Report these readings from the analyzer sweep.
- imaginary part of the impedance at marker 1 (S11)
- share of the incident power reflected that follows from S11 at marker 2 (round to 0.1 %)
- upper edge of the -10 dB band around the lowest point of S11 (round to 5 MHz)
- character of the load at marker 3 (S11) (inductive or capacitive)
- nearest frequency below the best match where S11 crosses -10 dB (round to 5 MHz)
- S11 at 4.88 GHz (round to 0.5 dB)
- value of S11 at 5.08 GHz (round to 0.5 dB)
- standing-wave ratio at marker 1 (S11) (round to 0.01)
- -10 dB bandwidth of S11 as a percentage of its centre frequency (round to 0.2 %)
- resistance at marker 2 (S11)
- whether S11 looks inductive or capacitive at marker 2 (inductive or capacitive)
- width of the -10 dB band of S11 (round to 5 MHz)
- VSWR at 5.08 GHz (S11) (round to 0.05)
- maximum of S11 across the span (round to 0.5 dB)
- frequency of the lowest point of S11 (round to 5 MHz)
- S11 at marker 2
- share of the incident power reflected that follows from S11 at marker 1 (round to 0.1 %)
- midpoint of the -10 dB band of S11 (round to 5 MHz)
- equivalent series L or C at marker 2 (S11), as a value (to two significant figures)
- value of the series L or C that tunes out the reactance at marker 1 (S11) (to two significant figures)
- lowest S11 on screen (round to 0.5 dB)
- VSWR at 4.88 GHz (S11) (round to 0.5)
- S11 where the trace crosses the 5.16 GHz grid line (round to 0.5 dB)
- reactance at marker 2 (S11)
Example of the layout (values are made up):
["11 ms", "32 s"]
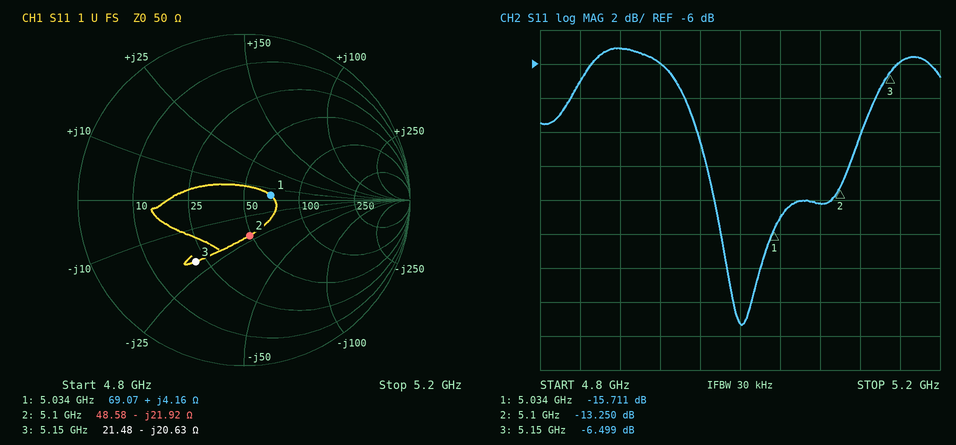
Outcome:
["+4.16 Ω", "4.7 %", "5.120 GHz", "capacitive", "4.955 GHz", "-5.0 dB", "-14.0 dB", "1.39", "3.2 %", "48.58 Ω", "capacitive", "165 MHz", "1.50", "-5.0 dB", "5.000 GHz", "-13.250 dB", "2.7 %", "5.040 GHz", "1.4 pF", "7.6 pF", "-21.5 dB", "3.5", "-6.0 dB", "-21.92 Ω"]
